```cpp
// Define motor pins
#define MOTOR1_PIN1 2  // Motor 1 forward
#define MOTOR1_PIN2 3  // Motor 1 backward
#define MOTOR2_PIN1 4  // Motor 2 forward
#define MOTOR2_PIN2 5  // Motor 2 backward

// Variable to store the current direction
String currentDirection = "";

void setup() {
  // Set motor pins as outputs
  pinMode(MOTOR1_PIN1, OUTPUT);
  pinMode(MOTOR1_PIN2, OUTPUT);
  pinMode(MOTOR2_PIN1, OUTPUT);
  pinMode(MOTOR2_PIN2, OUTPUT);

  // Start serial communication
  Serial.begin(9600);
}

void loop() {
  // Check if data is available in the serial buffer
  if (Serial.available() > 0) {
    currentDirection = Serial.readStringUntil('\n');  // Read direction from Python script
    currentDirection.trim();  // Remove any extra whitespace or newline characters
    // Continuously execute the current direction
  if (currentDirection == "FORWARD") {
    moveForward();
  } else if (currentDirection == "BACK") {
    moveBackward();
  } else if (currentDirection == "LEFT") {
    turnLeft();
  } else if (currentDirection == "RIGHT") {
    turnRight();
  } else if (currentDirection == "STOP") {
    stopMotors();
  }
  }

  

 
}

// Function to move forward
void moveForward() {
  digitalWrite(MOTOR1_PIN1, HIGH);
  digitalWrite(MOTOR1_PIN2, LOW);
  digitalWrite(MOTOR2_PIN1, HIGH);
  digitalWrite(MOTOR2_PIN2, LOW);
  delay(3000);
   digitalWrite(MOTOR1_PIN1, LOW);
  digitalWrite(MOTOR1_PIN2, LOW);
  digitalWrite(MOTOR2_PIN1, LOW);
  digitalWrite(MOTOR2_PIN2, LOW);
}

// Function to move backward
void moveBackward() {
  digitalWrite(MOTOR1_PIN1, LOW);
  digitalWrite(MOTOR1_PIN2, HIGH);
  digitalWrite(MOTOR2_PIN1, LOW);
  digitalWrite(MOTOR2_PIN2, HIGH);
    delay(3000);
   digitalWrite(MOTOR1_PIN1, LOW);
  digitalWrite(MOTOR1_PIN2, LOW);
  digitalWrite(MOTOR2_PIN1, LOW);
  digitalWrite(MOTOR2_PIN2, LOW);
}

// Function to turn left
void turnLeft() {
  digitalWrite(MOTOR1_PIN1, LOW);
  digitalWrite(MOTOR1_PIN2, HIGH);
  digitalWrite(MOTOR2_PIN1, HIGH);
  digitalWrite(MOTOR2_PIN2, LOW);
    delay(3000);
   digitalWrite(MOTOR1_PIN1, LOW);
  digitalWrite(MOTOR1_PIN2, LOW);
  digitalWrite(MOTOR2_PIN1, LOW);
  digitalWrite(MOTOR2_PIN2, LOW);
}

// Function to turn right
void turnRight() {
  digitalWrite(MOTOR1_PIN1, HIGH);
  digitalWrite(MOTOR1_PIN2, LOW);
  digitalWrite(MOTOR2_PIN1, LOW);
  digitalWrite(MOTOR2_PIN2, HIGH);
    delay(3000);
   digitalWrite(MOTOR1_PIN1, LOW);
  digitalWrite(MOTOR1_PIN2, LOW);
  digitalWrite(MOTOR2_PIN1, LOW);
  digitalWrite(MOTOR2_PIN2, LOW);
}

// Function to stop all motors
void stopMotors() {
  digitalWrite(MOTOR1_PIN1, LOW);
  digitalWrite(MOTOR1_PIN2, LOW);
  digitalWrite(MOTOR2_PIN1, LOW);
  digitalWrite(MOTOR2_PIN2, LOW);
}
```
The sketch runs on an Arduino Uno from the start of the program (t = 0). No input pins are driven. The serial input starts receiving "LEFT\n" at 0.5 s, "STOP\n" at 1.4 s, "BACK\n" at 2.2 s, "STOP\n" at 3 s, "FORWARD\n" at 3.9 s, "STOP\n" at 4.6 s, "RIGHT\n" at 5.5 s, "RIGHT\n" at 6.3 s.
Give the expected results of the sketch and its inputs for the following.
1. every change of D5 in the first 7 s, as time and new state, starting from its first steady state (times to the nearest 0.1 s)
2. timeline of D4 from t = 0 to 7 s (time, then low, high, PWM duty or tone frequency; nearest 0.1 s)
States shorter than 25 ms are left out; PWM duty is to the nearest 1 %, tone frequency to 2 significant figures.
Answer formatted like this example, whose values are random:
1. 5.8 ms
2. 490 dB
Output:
1. 0 s low; 3.5 s high; 6.5 s low
2. 0 s low; 0.5 s high; 3.5 s low; 6.5 s high
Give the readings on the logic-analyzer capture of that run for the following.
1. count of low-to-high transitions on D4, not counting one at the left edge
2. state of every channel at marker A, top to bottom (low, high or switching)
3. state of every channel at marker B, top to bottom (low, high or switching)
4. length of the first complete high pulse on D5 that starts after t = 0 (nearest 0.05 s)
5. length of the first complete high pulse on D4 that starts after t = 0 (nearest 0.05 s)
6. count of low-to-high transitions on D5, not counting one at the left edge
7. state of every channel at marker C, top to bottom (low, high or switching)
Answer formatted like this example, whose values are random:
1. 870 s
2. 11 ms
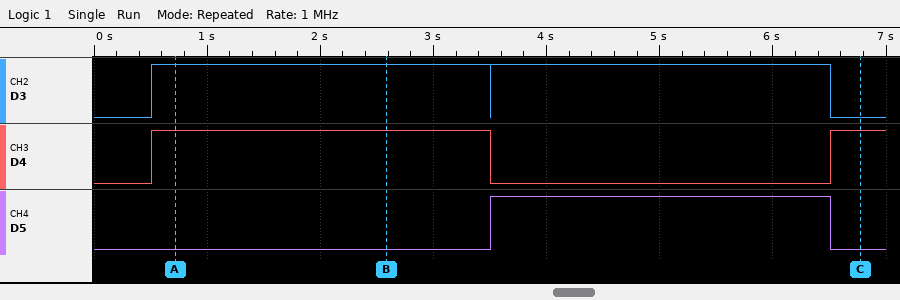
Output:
1. 2
2. D3 high, D4 high, D5 low
3. D3 high, D4 high, D5 low
4. 3.00 s
5. 3.00 s
6. 1
7. D3 low, D4 high, D5 low
